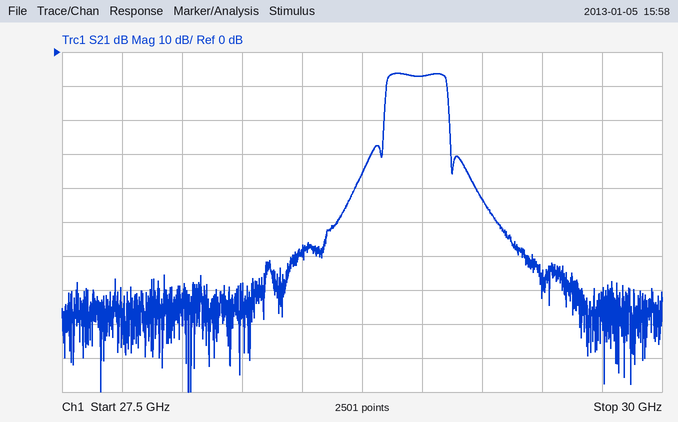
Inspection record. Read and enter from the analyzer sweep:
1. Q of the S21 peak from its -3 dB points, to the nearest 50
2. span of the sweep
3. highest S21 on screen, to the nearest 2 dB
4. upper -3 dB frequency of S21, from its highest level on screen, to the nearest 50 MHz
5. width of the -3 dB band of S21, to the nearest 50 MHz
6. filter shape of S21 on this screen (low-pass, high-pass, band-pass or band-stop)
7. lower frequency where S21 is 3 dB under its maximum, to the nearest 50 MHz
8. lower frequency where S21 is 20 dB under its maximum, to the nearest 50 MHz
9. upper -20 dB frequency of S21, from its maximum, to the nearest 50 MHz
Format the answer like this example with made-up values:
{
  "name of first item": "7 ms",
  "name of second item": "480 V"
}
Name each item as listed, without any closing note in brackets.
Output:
{
  "Q of the S21 peak from its -3 dB points, to the nearest 50": "100",
  "span of the sweep": "2.5 GHz",
  "highest S21 on screen, to the nearest 2 dB": "-6 dB",
  "upper -3 dB frequency of S21, from its highest level on screen, to the nearest 50 MHz": "29.10 GHz",
  "width of the -3 dB band of S21, to the nearest 50 MHz": "250 MHz",
  "filter shape of S21 on this screen": "band-pass",
  "lower frequency where S21 is 3 dB under its maximum, to the nearest 50 MHz": "28.85 GHz",
  "lower frequency where S21 is 20 dB under its maximum, to the nearest 50 MHz": "28.85 GHz",
  "upper -20 dB frequency of S21, from its maximum, to the nearest 50 MHz": "29.10 GHz"
}
